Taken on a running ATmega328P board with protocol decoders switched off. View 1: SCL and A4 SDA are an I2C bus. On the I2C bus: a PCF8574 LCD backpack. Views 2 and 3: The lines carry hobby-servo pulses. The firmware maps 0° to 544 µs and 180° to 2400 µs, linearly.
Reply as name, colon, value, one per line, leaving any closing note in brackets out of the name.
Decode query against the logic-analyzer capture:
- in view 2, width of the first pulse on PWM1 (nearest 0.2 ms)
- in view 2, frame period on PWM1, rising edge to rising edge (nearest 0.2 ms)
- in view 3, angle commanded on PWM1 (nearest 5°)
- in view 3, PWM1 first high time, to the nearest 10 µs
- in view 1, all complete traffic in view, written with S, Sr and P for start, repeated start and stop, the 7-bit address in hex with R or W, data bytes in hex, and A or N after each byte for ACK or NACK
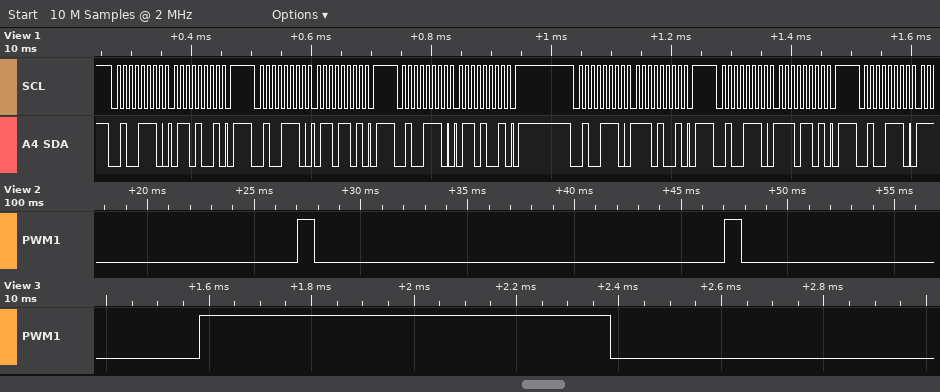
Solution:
in view 2, width of the first pulse on PWM1: 0.8 ms
in view 2, frame period on PWM1, rising edge to rising edge: 20.0 ms
in view 3, angle commanded on PWM1: 25°
in view 3, PWM1 first high time, to the nearest 10 µs: 800 µs
in view 1, all complete traffic in view, written with S, Sr and P for start, repeated start and stop, the 7-bit address in hex with R or W, data bytes in hex, and A or N after each byte for ACK or NACK: S 27W A 69 A P S 27W A 6D A P S 27W A 69 A P S 27W A E9 A P S 27W A ED A P S 27W A
